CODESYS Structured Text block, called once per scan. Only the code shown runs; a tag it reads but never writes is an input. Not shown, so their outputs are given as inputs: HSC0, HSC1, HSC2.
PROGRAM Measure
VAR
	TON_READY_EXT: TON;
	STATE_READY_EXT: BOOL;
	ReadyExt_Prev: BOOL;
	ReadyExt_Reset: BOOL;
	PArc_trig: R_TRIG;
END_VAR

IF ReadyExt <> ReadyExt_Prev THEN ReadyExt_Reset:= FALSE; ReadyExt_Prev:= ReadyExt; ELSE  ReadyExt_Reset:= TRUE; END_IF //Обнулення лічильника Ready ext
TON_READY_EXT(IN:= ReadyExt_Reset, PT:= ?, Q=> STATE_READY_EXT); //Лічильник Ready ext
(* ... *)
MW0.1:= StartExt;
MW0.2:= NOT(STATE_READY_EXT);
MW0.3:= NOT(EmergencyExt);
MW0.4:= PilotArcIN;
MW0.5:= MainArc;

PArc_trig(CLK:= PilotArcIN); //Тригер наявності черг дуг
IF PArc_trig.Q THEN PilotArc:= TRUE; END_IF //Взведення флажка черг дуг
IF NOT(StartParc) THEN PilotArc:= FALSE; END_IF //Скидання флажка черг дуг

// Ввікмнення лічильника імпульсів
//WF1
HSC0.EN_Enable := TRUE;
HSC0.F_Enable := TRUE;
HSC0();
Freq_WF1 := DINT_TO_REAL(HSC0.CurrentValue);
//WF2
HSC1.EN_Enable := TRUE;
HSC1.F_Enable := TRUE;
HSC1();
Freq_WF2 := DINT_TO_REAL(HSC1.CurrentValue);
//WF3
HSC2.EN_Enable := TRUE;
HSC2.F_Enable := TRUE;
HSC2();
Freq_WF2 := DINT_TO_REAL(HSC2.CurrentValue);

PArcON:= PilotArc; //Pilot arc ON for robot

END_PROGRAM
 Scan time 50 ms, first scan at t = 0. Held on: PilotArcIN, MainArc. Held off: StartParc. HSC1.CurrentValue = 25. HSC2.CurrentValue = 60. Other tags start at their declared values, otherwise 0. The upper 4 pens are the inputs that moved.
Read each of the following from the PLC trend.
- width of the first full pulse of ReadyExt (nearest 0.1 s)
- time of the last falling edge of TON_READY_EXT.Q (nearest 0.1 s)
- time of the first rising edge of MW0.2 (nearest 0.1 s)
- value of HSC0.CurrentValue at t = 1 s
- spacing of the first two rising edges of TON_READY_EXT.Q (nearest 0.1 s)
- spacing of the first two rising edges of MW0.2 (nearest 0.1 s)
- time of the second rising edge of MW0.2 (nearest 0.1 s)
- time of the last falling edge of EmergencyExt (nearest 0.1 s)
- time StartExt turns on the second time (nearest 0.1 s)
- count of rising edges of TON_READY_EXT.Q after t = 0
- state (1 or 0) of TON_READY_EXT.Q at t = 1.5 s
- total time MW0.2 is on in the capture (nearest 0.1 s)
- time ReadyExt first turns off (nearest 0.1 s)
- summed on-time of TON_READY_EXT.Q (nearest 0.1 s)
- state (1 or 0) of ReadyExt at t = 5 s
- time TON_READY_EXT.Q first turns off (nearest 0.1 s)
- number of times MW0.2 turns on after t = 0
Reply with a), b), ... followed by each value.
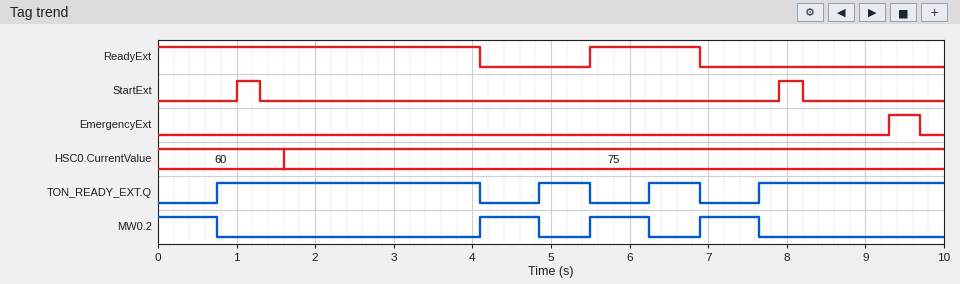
a) 1.4 s
b) 6.9 s
c) 4.1 s
d) 60
e) 4.1 s
f) 1.4 s
g) 5.5 s
h) 9.7 s
i) 7.9 s
j) 4
k) 1
l) 3.0 s
m) 4.1 s
n) 7.0 s
o) 0
p) 4.1 s
q) 3
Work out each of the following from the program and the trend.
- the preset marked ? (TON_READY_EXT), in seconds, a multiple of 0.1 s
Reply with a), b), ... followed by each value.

a) 0.7 s
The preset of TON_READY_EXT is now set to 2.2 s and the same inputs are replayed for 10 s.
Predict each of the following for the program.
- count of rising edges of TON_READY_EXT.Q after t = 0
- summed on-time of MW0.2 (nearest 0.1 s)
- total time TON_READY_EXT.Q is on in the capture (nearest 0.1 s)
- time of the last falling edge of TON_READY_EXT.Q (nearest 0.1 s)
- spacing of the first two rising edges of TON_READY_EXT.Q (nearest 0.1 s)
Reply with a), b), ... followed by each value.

a) 2
b) 7.3 s
c) 2.7 s
d) 4.1 s
e) 6.9 s
